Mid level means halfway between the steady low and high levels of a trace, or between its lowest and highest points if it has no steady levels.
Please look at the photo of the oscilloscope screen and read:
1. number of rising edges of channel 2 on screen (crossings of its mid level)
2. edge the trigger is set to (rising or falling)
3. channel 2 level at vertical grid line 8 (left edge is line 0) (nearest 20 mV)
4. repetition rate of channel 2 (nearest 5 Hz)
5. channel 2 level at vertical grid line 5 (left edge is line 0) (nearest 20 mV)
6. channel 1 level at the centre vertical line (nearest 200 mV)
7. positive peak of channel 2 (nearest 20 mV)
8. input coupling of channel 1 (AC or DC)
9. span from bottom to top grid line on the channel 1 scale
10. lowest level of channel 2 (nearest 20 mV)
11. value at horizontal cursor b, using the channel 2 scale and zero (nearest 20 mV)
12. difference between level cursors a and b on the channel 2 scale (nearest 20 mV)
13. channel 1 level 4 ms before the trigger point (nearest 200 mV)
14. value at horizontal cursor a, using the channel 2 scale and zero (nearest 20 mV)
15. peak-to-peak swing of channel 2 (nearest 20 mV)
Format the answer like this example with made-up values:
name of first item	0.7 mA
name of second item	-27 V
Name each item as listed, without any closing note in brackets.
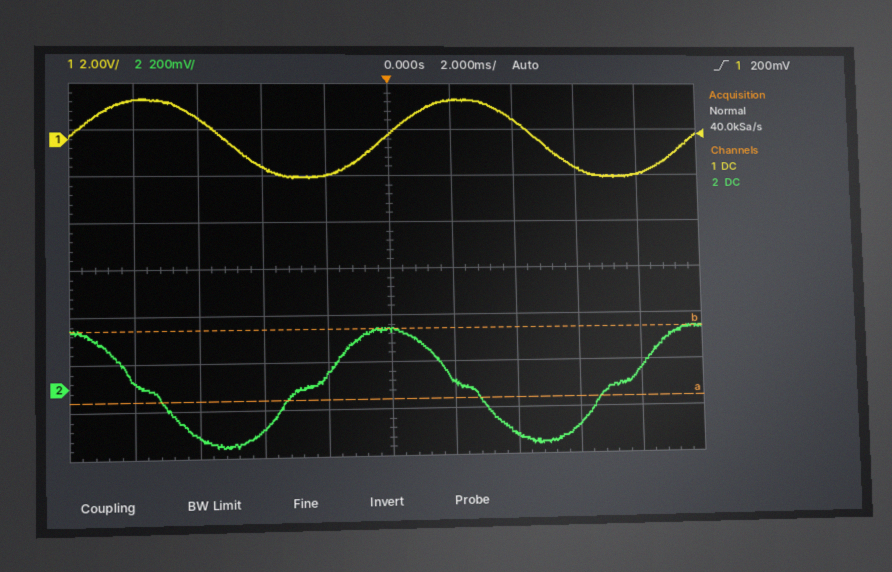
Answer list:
number of rising edges of channel 2 on screen	2
edge the trigger is set to	rising
channel 2 level at vertical grid line 8 (left edge is line 0)	-180 mV
repetition rate of channel 2	100 Hz
channel 2 level at vertical grid line 5 (left edge is line 0)	240 mV
channel 1 level at the centre vertical line	200 mV
positive peak of channel 2	240 mV
input coupling of channel 1	DC
span from bottom to top grid line on the channel 1 scale	16 V
lowest level of channel 2	-260 mV
value at horizontal cursor b, using the channel 2 scale and zero	240 mV
difference between level cursors a and b on the channel 2 scale	300 mV
channel 1 level 4 ms before the trigger point	-1.2 V
value at horizontal cursor a, using the channel 2 scale and zero	-60 mV
peak-to-peak swing of channel 2	500 mV
